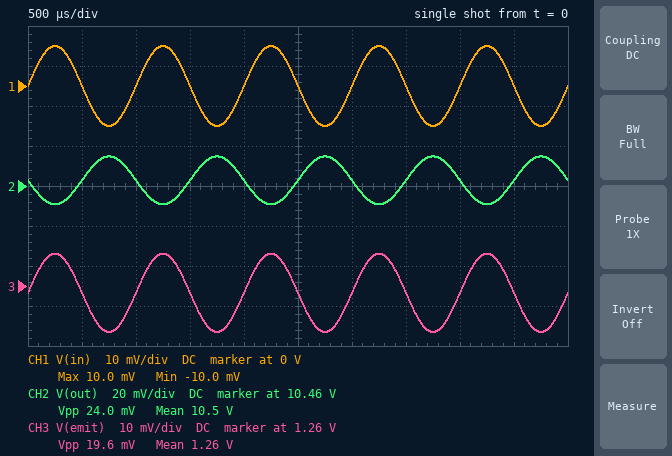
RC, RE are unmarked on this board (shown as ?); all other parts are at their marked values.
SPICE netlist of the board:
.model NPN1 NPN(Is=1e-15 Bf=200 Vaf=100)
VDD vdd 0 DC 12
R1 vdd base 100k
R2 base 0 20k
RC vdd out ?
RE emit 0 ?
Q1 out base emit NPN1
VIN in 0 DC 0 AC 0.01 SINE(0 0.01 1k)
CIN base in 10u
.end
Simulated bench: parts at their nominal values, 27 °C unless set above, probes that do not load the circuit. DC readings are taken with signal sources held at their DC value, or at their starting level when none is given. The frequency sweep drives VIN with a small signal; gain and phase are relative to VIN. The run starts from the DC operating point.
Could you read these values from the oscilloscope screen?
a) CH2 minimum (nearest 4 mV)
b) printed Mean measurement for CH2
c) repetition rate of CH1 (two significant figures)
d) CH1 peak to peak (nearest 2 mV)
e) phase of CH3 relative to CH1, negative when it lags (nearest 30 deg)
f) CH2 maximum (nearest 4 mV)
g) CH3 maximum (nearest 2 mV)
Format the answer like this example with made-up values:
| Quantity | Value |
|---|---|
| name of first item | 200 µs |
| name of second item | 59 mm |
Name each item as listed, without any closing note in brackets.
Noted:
| Quantity | Value |
|---|---|
| CH2 minimum | 10.452 V |
| printed Mean measurement for CH2 | 10.5 V |
| repetition rate of CH1 | 1.0 kHz |
| CH1 peak to peak | 20 mV |
| phase of CH3 relative to CH1, negative when it lags | 0 deg |
| CH2 maximum | 10.476 V |
| CH3 maximum | 1.268 V |
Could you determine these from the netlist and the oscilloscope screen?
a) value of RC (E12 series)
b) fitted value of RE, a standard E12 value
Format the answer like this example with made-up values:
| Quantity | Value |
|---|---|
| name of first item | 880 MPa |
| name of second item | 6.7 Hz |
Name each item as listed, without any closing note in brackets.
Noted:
| Quantity | Value |
|---|---|
| value of RC | 2.7 kΩ |
| fitted value of RE, a standard E12 value | 2.2 kΩ |
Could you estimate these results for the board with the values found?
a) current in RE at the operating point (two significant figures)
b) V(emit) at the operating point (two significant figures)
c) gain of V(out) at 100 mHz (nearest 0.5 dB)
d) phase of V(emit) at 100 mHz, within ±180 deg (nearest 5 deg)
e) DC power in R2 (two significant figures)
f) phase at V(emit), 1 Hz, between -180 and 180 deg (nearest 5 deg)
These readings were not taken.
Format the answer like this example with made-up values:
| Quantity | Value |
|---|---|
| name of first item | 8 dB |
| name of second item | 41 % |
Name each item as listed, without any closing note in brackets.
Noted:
| Quantity | Value |
|---|---|
| current in RE at the operating point | 570 µA |
| V(emit) at the operating point | 1.3 V |
| gain of V(out) at 100 mHz | -18.5 dB |
| phase of V(emit) at 100 mHz, within ±180 deg | 85 deg |
| DC power in R2 | 190 µW |
| phase at V(emit), 1 Hz, between -180 and 180 deg | 45 deg |
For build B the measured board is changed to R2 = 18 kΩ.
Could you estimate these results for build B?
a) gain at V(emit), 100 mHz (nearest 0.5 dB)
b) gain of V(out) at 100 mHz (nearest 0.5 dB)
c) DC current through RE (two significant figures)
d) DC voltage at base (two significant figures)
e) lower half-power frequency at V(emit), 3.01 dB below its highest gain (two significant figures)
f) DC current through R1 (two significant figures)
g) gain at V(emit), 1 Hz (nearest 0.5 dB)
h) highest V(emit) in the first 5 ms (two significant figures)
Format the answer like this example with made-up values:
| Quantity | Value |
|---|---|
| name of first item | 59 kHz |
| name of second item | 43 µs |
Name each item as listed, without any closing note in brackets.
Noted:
| Quantity | Value |
|---|---|
| gain at V(emit), 100 mHz | -21.0 dB |
| gain of V(out) at 100 mHz | -19.0 dB |
| DC current through RE | 500 µA |
| DC voltage at base | 1.8 V |
| lower half-power frequency at V(emit), 3.01 dB below its highest gain | 1.1 Hz |
| DC current through R1 | 100 µA |
| gain at V(emit), 1 Hz | -3.5 dB |
| highest V(emit) in the first 5 ms | 1.1 V |
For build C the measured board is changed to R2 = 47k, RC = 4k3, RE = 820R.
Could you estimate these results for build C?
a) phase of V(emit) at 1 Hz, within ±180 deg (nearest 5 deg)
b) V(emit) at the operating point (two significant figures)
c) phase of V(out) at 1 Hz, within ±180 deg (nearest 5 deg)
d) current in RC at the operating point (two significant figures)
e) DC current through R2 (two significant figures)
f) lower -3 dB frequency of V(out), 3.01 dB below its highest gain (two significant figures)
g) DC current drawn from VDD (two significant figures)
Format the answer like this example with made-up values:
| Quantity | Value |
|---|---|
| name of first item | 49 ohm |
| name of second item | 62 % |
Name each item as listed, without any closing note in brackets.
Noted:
| Quantity | Value |
|---|---|
| phase of V(emit) at 1 Hz, within ±180 deg | 85 deg |
| V(emit) at the operating point | 1.9 V |
| phase of V(out) at 1 Hz, within ±180 deg | -95 deg |
| current in RC at the operating point | 2.3 mA |
| DC current through R2 | 57 µA |
| lower -3 dB frequency of V(out), 3.01 dB below its highest gain | 19 Hz |
| DC current drawn from VDD | 2.4 mA |
